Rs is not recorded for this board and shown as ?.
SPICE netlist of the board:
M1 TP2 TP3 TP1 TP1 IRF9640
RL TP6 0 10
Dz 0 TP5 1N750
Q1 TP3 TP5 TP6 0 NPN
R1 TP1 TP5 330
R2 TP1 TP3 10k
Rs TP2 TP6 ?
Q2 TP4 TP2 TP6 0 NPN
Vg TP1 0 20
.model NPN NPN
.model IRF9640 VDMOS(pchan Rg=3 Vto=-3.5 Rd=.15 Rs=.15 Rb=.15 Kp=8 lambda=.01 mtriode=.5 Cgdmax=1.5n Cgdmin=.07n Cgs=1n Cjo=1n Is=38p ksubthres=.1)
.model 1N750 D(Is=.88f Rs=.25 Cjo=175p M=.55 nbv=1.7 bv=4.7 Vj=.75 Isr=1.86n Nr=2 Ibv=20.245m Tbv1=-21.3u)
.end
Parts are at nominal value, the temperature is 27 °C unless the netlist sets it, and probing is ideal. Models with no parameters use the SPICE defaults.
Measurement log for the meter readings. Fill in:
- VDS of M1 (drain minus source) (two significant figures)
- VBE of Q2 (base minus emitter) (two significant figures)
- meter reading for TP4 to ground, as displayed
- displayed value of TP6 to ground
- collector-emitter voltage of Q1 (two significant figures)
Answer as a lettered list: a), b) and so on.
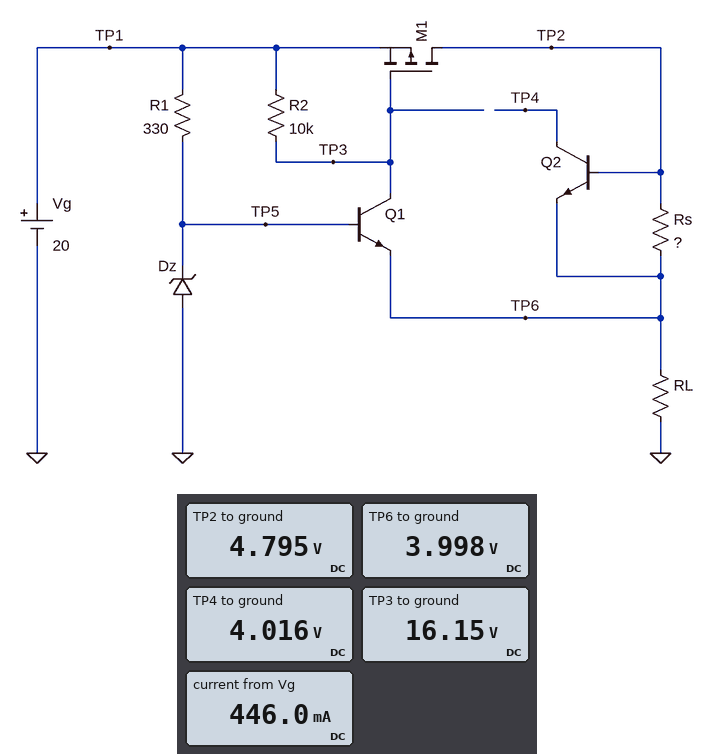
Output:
a) -15 V
b) 800 mV
c) 4.016 V
d) 3.998 V
e) 12 V
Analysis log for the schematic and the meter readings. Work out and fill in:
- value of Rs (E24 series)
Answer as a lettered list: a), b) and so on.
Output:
a) 2 Ω
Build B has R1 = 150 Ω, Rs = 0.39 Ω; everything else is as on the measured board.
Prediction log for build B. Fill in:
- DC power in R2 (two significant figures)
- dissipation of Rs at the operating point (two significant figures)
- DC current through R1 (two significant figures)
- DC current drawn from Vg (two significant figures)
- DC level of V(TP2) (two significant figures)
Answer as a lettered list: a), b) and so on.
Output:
a) 1.5 mW
b) 64 mW
c) 100 mA
d) 510 mA
e) 4.2 V
